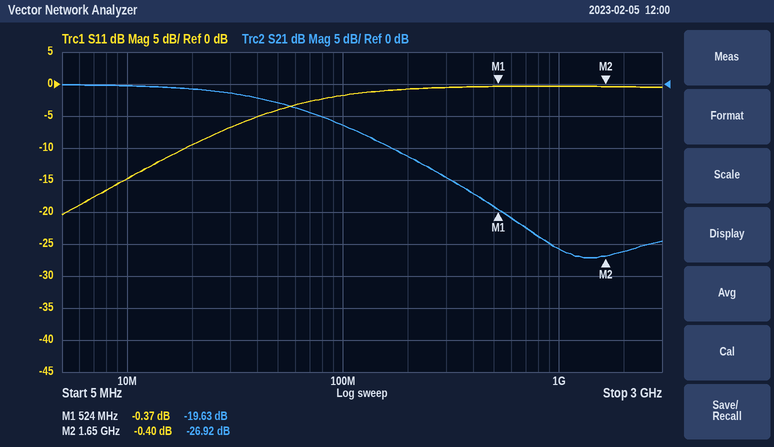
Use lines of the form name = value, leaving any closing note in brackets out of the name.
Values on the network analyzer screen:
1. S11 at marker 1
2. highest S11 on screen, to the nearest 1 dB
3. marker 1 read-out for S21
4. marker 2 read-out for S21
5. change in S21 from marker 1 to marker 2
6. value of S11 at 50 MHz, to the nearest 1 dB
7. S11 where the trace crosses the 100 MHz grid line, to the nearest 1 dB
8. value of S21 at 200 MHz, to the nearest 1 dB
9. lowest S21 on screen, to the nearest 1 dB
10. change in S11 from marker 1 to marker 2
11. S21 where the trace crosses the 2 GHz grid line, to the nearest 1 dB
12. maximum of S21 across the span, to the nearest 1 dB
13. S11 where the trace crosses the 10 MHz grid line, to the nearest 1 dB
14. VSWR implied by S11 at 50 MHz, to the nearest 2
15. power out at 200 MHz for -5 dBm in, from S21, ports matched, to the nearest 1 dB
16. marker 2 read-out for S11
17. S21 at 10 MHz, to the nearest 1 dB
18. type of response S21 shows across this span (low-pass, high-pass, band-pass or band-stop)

S11 at marker 1 = -0.37 dB
highest S11 on screen, to the nearest 1 dB = 0 dB
marker 1 read-out for S21 = -19.63 dB
marker 2 read-out for S21 = -26.92 dB
change in S21 from marker 1 to marker 2 = -7.29 dB
value of S11 at 50 MHz, to the nearest 1 dB = -4 dB
S11 where the trace crosses the 100 MHz grid line, to the nearest 1 dB = -2 dB
value of S21 at 200 MHz, to the nearest 1 dB = -11 dB
lowest S21 on screen, to the nearest 1 dB = -27 dB
change in S11 from marker 1 to marker 2 = -0.03 dB
S21 where the trace crosses the 2 GHz grid line, to the nearest 1 dB = -26 dB
maximum of S21 across the span, to the nearest 1 dB = 0 dB
S11 where the trace crosses the 10 MHz grid line, to the nearest 1 dB = -15 dB
VSWR implied by S11 at 50 MHz, to the nearest 2 = 4
power out at 200 MHz for -5 dBm in, from S21, ports matched, to the nearest 1 dB = -16 dBm
marker 2 read-out for S11 = -0.40 dB
S21 at 10 MHz, to the nearest 1 dB = 0 dB
type of response S21 shows across this span = low-pass
